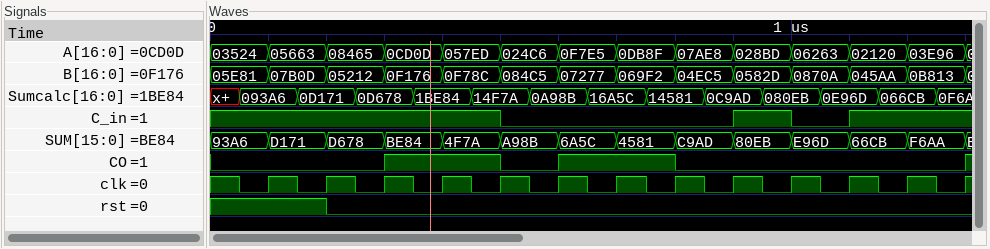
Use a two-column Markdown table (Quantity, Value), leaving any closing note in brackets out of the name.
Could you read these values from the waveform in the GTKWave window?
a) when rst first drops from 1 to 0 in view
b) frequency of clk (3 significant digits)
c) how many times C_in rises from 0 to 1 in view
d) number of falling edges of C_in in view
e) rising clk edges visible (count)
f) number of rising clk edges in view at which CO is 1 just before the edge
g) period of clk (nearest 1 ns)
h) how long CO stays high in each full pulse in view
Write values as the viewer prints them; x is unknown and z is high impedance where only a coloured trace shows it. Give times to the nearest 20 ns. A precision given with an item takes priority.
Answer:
| Quantity | Value |
|---|---|
| when rst first drops from 1 to 0 in view | 200 ns |
| frequency of clk | 10.0 MHz |
| how many times C_in rises from 0 to 1 in view | 2 |
| number of falling edges of C_in in view | 2 |
| rising clk edges visible | 13 |
| number of rising clk edges in view at which CO is 1 just before the edge | 4 |
| period of clk | 100 ns |
| how long CO stays high in each full pulse in view | 200 ns, 200 ns |
